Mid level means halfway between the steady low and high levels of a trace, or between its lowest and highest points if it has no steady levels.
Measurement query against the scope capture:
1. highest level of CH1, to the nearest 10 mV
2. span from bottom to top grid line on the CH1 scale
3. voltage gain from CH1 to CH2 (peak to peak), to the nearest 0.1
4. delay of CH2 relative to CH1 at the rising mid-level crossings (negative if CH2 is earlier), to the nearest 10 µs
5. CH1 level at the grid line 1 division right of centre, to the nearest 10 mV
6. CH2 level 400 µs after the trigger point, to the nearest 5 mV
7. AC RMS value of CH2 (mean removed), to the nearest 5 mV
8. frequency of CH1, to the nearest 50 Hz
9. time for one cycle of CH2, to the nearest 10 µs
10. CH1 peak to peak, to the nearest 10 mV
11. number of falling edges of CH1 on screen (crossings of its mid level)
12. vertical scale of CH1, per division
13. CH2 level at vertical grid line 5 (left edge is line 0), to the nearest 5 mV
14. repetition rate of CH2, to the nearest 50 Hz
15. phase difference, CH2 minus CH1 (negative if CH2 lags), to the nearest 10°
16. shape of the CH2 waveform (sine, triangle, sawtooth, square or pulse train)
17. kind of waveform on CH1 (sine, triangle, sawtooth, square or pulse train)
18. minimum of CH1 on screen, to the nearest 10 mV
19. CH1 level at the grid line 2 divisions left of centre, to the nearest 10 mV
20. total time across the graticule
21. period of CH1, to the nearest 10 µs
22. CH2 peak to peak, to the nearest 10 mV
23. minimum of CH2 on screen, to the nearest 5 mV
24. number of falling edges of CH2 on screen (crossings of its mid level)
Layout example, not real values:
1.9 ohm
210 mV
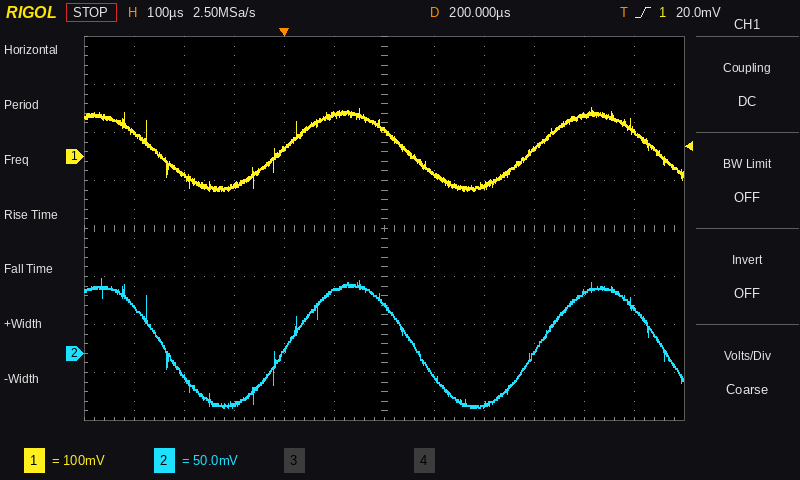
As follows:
100 mV
800 mV
0.8
+10 µs
-40 mV
-55 mV
45 mV
2.00 kHz
500 µs
170 mV
3
100 mV
65 mV
2.00 kHz
-10°
sine
sine
-70 mV
20 mV
1.2 ms
500 µs
130 mV
-55 mV
3
